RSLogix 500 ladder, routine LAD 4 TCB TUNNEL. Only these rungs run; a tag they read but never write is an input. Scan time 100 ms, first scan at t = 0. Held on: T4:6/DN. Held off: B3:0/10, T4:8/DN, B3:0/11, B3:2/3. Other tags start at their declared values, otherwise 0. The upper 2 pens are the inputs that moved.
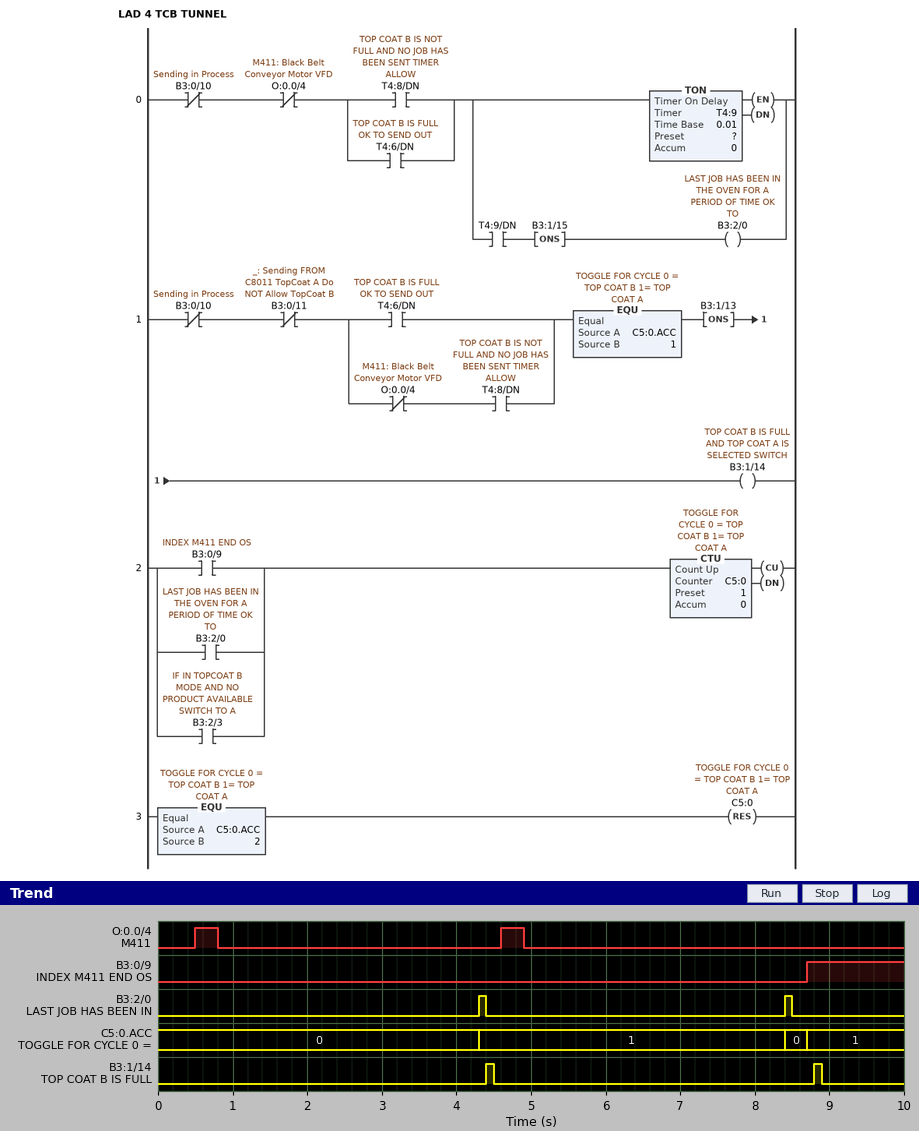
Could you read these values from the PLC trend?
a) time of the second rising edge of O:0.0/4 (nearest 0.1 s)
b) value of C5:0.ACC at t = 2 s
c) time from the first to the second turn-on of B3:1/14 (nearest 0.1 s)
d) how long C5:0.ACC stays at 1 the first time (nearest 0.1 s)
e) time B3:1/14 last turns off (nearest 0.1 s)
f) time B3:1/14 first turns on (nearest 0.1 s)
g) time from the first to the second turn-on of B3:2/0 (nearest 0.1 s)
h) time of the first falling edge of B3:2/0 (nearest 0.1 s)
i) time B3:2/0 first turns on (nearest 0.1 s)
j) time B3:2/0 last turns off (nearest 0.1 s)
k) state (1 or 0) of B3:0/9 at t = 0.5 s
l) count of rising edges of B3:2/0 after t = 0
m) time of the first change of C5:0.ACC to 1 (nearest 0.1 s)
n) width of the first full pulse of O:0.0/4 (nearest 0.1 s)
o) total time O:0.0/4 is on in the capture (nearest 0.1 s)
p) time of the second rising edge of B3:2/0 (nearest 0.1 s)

4.6 s
0
4.4 s
4.1 s
8.9 s
4.4 s
4.1 s
4.4 s
4.3 s
8.5 s
0
2
4.3 s
0.3 s
0.6 s
8.4 s
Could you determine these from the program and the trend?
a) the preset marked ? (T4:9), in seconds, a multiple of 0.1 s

3.5 s
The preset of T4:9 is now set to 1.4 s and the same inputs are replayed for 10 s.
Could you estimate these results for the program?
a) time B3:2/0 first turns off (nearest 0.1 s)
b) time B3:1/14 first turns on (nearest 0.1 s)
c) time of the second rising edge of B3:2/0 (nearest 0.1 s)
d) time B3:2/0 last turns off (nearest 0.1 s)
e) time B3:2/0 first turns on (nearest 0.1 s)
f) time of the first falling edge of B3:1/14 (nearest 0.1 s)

2.3 s
2.3 s
6.3 s
6.4 s
2.2 s
2.4 s
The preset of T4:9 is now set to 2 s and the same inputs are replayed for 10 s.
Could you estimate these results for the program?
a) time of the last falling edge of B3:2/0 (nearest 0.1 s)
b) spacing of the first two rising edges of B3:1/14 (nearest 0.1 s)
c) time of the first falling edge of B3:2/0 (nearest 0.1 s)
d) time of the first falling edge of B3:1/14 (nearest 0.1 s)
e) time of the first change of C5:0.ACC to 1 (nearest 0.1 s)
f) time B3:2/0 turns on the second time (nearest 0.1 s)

7.0 s
5.9 s
2.9 s
3.0 s
2.8 s
6.9 s
